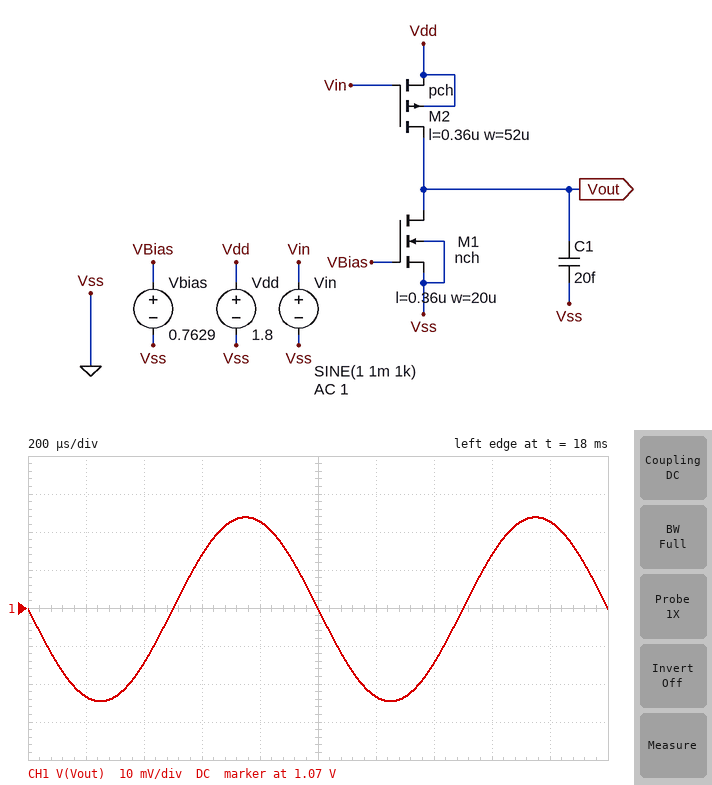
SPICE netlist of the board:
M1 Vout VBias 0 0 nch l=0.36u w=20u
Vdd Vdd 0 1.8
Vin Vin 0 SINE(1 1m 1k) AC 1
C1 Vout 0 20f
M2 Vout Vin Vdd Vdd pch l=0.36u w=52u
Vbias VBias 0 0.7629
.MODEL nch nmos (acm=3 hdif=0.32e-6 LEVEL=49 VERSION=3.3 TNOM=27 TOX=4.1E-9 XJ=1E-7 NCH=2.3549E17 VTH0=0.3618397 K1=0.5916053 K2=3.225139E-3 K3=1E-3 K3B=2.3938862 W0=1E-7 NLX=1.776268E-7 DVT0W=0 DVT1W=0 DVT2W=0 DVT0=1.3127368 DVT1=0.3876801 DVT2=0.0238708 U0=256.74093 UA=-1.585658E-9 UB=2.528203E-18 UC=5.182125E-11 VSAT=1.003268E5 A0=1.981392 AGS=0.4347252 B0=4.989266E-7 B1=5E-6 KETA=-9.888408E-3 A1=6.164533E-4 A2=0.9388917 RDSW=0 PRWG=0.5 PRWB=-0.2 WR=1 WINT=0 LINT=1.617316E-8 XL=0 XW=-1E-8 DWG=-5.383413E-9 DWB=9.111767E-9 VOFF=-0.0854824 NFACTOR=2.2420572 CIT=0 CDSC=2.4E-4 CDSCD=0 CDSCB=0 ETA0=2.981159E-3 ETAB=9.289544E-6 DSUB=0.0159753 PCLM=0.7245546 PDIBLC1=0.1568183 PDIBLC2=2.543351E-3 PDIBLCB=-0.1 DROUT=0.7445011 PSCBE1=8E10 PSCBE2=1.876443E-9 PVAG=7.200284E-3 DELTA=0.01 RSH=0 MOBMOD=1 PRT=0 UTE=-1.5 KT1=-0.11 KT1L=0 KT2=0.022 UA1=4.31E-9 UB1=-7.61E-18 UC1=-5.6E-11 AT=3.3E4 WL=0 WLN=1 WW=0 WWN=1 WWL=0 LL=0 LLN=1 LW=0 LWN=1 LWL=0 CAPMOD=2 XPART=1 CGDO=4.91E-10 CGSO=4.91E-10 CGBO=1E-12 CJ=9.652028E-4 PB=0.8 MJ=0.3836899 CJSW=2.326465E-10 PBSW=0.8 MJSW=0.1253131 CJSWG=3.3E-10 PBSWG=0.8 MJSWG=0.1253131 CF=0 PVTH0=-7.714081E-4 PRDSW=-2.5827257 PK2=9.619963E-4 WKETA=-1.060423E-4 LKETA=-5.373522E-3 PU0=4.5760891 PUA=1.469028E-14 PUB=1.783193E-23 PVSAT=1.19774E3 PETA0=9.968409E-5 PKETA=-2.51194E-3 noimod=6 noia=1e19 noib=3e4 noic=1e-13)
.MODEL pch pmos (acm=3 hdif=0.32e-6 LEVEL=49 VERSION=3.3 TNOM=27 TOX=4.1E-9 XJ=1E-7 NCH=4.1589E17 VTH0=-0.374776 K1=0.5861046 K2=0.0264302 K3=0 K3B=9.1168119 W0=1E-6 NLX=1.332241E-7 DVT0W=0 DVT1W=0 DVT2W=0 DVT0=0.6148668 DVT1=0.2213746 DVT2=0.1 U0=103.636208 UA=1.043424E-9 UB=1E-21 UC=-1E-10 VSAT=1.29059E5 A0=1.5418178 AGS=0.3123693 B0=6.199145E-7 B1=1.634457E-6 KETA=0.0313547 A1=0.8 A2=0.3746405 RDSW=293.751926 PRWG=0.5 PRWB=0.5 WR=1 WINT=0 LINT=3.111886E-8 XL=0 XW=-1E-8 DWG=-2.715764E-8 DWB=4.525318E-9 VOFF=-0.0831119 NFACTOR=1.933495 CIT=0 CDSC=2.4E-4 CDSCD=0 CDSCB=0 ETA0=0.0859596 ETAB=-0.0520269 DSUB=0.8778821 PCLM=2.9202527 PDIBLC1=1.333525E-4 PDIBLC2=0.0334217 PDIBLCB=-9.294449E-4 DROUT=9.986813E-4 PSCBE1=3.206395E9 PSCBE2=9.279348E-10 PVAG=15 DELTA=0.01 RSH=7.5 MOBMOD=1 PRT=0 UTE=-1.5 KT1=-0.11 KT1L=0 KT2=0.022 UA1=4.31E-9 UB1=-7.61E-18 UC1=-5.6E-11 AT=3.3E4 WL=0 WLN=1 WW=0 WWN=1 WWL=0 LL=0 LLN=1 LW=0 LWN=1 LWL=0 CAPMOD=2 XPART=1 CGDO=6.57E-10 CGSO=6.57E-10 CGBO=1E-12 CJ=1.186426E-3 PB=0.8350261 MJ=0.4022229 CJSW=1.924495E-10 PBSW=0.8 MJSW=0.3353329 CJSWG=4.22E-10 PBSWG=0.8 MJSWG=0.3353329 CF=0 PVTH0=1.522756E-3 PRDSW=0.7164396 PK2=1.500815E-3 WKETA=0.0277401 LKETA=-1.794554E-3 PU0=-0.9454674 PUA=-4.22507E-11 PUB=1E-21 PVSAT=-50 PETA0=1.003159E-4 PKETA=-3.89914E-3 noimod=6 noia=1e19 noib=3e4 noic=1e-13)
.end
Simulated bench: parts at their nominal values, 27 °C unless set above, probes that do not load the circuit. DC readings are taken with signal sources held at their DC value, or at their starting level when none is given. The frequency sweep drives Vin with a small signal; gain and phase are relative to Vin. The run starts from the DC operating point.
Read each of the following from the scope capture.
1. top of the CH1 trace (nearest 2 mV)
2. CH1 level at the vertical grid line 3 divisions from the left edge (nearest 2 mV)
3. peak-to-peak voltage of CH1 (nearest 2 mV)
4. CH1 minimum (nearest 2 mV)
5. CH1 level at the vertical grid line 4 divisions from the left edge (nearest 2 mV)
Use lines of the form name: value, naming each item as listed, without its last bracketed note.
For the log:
top of the CH1 trace: 1.094 V
CH1 level at the vertical grid line 3 divisions from the left edge: 1.084 V
peak-to-peak voltage of CH1: 48 mV
CH1 minimum: 1.046 V
CH1 level at the vertical grid line 4 divisions from the left edge: 1.092 V
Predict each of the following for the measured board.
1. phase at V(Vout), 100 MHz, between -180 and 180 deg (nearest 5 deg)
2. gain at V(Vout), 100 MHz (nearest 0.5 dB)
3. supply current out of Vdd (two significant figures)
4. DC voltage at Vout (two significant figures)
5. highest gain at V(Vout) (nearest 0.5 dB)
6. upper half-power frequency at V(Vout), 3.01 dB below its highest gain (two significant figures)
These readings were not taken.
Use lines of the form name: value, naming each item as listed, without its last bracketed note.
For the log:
phase at V(Vout), 100 MHz, between -180 and 180 deg: 145 deg
gain at V(Vout), 100 MHz: 26.0 dB
supply current out of Vdd: 630 µA
DC voltage at Vout: 1.1 V
highest gain at V(Vout): 27.5 dB
upper half-power frequency at V(Vout), 3.01 dB below its highest gain: 150 MHz
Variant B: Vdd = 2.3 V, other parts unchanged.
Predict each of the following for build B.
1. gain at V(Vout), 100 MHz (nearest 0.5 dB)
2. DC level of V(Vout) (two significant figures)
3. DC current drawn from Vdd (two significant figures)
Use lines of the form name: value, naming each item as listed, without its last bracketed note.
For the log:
gain at V(Vout), 100 MHz: -20.5 dB
DC level of V(Vout): 2.2 V
DC current drawn from Vdd: 680 µA
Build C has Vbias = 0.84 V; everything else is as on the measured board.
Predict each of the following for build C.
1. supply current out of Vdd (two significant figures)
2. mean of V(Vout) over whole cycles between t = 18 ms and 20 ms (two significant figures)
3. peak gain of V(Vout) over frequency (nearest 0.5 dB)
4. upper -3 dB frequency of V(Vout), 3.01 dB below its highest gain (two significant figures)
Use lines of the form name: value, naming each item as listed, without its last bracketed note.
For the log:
supply current out of Vdd: 690 µA
mean of V(Vout) over whole cycles between t = 18 ms and 20 ms: 160 mV
peak gain of V(Vout) over frequency: 3.0 dB
upper -3 dB frequency of V(Vout), 3.01 dB below its highest gain: 2.5 GHz
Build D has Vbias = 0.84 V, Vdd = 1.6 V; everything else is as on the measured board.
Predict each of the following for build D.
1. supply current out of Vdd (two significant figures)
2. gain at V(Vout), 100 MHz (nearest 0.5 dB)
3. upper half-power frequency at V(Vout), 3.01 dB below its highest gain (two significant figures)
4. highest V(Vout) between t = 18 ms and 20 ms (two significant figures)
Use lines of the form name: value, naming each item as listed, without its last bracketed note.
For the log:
supply current out of Vdd: 150 µA
gain at V(Vout), 100 MHz: -10.0 dB
upper half-power frequency at V(Vout), 3.01 dB below its highest gain: 6.5 GHz
highest V(Vout) between t = 18 ms and 20 ms: 25 mV
